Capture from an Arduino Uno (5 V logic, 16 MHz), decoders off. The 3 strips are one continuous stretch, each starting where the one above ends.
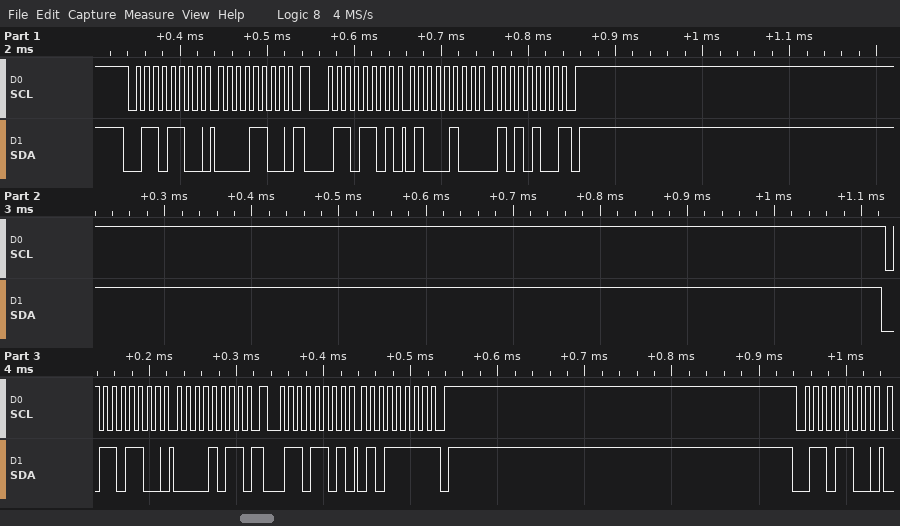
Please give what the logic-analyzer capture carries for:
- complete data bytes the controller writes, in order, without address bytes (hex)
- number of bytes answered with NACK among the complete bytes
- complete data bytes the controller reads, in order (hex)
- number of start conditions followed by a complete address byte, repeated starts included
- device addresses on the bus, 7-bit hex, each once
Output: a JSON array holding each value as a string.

["0C 0B", "2", "44 54 5F", "5", "0x36"]
